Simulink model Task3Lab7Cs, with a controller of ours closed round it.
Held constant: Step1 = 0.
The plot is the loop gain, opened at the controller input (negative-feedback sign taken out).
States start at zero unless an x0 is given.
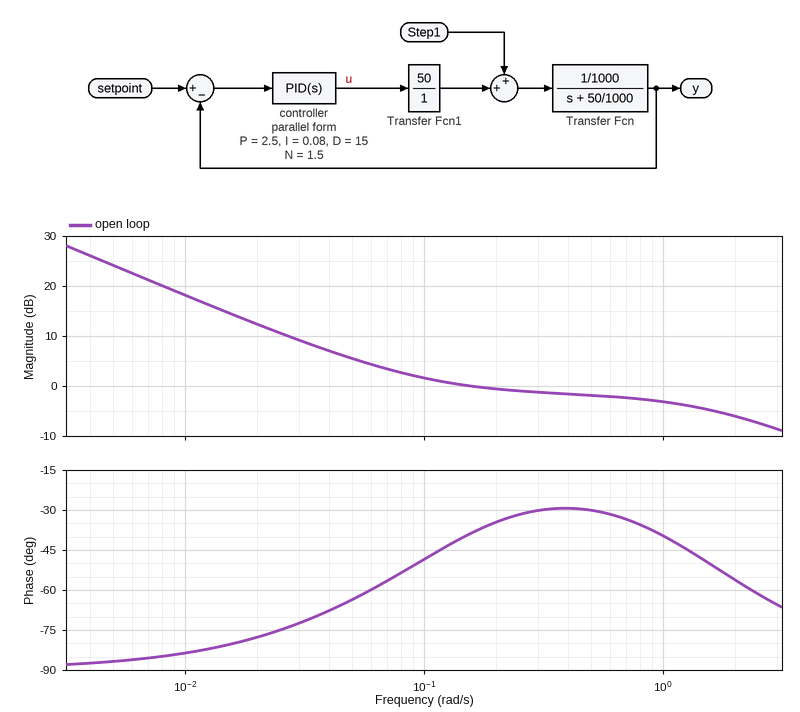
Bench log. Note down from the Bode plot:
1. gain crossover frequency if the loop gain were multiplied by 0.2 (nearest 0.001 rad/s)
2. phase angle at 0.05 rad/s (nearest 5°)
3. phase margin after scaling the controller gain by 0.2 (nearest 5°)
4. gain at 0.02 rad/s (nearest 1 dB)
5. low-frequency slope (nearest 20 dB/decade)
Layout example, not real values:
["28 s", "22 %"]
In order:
["0.016 rad/s", "-65°", "100°", "12 dB", "-20 dB/decade"]
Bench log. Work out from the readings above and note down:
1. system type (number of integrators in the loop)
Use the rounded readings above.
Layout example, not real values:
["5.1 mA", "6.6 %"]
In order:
["1"]
